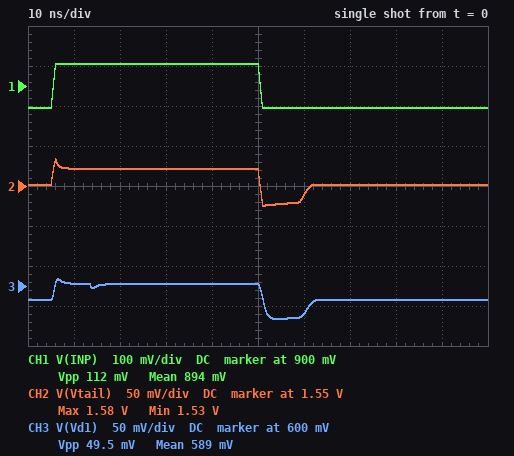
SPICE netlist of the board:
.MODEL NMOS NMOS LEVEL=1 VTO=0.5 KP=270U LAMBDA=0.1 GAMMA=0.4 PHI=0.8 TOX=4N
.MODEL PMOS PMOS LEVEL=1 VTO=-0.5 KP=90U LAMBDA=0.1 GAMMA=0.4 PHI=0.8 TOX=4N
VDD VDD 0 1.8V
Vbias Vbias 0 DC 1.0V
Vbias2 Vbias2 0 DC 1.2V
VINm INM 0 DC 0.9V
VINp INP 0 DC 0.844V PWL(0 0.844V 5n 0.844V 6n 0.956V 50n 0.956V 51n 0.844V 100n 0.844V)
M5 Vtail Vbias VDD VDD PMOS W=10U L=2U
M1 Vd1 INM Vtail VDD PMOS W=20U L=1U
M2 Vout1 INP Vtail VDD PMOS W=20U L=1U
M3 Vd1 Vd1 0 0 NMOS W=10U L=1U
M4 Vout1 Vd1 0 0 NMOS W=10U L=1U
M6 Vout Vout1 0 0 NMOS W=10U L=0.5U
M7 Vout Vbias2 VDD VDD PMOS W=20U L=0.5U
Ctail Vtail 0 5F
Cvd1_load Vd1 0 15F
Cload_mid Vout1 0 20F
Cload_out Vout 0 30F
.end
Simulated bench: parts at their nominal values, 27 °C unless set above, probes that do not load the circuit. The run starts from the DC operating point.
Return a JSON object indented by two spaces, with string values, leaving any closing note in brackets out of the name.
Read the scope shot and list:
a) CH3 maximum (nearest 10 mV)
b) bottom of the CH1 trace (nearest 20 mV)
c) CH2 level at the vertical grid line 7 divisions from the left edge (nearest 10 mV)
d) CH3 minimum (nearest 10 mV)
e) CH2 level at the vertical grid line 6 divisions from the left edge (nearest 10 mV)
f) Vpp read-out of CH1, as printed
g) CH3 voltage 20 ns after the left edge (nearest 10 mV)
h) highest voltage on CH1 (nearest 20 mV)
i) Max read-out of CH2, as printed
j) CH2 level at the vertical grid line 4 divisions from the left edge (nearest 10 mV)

{
  "CH3 maximum": "610 mV",
  "bottom of the CH1 trace": "840 mV",
  "CH2 level at the vertical grid line 7 divisions from the left edge": "1.55 V",
  "CH3 minimum": "560 mV",
  "CH2 level at the vertical grid line 6 divisions from the left edge": "1.54 V",
  "Vpp read-out of CH1, as printed": "112 mV",
  "CH3 voltage 20 ns after the left edge": "600 mV",
  "highest voltage on CH1": "960 mV",
  "Max read-out of CH2, as printed": "1.58 V",
  "CH2 level at the vertical grid line 4 divisions from the left edge": "1.57 V"
}
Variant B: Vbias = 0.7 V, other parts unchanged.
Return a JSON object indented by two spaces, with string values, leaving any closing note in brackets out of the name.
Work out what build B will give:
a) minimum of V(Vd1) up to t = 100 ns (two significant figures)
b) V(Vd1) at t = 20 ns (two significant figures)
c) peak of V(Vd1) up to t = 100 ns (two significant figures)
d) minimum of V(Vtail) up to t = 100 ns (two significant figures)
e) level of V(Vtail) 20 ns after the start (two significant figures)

{
  "minimum of V(Vd1) up to t = 100 ns": "610 mV",
  "V(Vd1) at t = 20 ns": "640 mV",
  "peak of V(Vd1) up to t = 100 ns": "650 mV",
  "minimum of V(Vtail) up to t = 100 ns": "1.6 V",
  "level of V(Vtail) 20 ns after the start": "1.6 V"
}
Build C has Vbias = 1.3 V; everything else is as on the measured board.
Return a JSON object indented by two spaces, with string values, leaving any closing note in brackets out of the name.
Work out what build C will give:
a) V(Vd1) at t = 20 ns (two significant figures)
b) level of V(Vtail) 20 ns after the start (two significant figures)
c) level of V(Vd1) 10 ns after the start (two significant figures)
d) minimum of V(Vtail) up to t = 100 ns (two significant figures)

{
  "V(Vd1) at t = 20 ns": "510 mV",
  "level of V(Vtail) 20 ns after the start": "1.5 V",
  "level of V(Vd1) 10 ns after the start": "520 mV",
  "minimum of V(Vtail) up to t = 100 ns": "1.4 V"
}
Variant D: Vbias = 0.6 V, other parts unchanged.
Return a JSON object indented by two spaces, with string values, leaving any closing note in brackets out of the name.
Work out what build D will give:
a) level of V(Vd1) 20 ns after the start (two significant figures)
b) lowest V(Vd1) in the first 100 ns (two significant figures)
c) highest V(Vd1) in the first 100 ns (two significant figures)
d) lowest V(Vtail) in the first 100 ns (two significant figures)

{
  "level of V(Vd1) 20 ns after the start": "650 mV",
  "lowest V(Vd1) in the first 100 ns": "620 mV",
  "highest V(Vd1) in the first 100 ns": "660 mV",
  "lowest V(Vtail) in the first 100 ns": "1.6 V"
}
